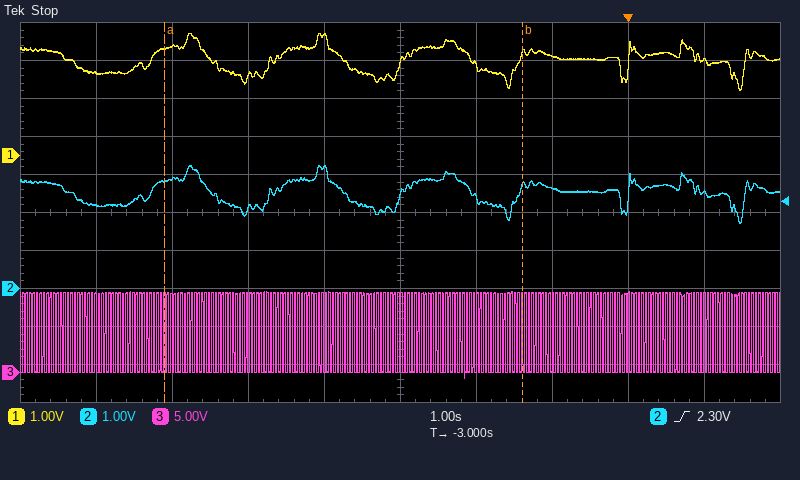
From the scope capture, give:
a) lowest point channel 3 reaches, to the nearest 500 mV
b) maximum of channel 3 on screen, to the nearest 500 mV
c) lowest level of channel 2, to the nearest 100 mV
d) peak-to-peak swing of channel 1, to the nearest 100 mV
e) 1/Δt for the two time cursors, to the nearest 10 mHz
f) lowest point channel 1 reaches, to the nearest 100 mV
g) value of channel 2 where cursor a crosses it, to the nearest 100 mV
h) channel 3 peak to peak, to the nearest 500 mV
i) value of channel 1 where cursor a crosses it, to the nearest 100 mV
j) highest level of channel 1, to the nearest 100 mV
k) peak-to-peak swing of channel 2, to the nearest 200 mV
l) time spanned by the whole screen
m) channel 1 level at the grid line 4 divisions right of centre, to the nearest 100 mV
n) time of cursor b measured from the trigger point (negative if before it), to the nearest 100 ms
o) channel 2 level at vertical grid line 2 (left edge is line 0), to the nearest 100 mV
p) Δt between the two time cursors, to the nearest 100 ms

-1.0 V
10.5 V
1.7 V
1.5 V
210 mHz
1.7 V
2.8 V
11.5 V
2.8 V
3.2 V
1.6 V
10 s
2.5 V
-1.4 s
2.9 V
4.7 s
